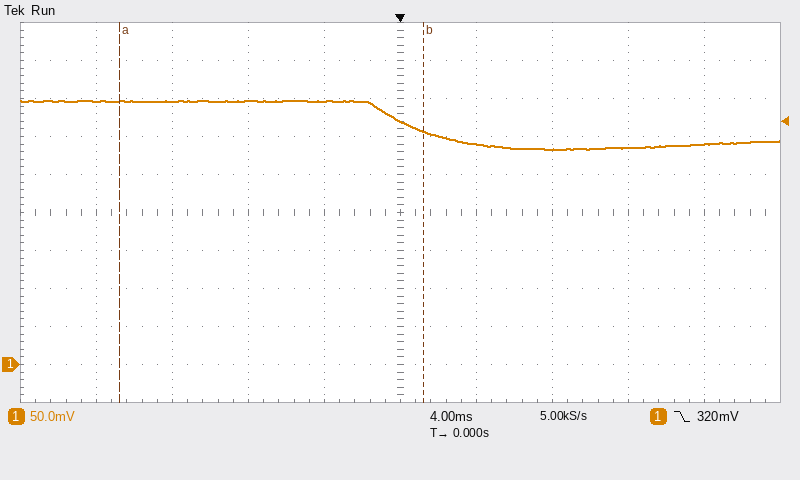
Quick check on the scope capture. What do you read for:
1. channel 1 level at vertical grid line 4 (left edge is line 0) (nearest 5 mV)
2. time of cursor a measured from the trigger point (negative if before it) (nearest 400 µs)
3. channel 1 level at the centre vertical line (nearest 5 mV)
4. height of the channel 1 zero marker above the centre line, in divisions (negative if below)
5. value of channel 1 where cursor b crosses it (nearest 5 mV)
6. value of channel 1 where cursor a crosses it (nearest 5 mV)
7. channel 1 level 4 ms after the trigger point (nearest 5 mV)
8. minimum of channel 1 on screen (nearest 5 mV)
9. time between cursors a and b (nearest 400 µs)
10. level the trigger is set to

345 mV
-14.8 ms
320 mV
-4.0 div
305 mV
345 mV
290 mV
285 mV
16.0 ms
320 mV
